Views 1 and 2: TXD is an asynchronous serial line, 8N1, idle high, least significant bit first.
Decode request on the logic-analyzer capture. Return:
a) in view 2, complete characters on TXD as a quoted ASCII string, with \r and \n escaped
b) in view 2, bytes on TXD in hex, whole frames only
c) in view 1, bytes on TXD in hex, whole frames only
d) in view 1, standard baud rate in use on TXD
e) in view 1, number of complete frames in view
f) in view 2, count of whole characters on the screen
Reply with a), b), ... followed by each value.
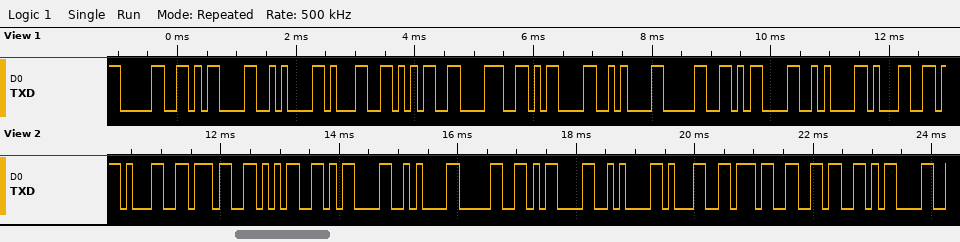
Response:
a) "175\r\n0\r\n176\r"
b) 31 37 35 0D 0A 30 0D 0A 31 37 36 0D
c) 30 0D 0A 31 35 38 0D 0A 30 0D 0A 31
d) 9600 baud
e) 12
f) 12
